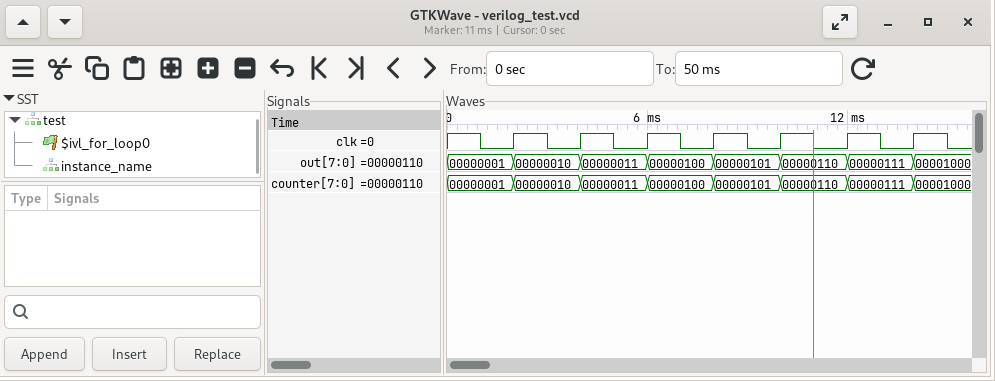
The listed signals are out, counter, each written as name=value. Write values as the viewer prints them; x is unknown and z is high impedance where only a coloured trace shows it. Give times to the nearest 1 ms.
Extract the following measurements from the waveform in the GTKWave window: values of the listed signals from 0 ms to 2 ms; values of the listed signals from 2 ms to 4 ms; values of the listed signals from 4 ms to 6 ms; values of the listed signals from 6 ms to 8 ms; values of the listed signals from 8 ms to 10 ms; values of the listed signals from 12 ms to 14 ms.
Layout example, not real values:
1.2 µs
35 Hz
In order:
out=00000001, counter=00000001
out=00000010, counter=00000010
out=00000011, counter=00000011
out=00000100, counter=00000100
out=00000101, counter=00000101
out=00000111, counter=00000111
